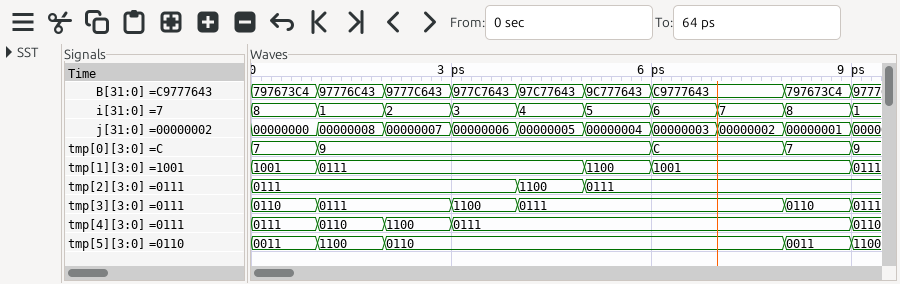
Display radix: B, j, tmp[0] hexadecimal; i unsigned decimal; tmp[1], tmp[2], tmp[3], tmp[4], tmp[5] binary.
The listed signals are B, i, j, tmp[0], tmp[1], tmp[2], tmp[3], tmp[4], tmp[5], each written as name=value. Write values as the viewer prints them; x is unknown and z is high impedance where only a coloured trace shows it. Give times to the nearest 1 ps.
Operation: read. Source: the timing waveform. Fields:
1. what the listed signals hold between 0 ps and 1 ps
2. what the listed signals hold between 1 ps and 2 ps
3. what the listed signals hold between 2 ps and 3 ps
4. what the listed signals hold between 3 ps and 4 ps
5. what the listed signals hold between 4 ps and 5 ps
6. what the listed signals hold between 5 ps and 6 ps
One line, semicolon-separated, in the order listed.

B=797673C4, i=8, j=00000000, tmp[0]=7, tmp[1]=1001, tmp[2]=0111, tmp[3]=0110, tmp[4]=0111, tmp[5]=0011; B=97776C43, i=1, j=00000008, tmp[0]=9, tmp[1]=0111, tmp[2]=0111, tmp[3]=0111, tmp[4]=0110, tmp[5]=1100; B=9777C643, i=2, j=00000007, tmp[0]=9, tmp[1]=0111, tmp[2]=0111, tmp[3]=0111, tmp[4]=1100, tmp[5]=0110; B=977C7643, i=3, j=00000006, tmp[0]=9, tmp[1]=0111, tmp[2]=0111, tmp[3]=1100, tmp[4]=0111, tmp[5]=0110; B=97C77643, i=4, j=00000005, tmp[0]=9, tmp[1]=0111, tmp[2]=1100, tmp[3]=0111, tmp[4]=0111, tmp[5]=0110; B=9C777643, i=5, j=00000004, tmp[0]=9, tmp[1]=1100, tmp[2]=0111, tmp[3]=0111, tmp[4]=0111, tmp[5]=0110
